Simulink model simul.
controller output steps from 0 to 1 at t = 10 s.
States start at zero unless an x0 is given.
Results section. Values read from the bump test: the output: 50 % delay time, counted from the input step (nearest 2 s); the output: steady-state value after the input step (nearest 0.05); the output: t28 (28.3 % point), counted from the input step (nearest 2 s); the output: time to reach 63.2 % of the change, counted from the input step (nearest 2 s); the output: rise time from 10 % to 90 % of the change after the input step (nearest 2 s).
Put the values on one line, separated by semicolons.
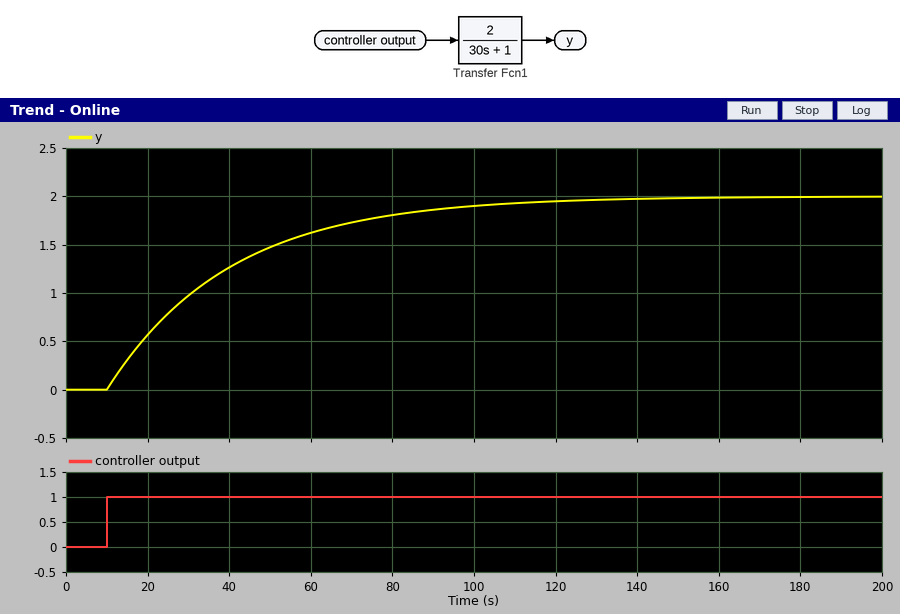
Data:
20 s; 2.00; 10 s; 30 s; 66 s
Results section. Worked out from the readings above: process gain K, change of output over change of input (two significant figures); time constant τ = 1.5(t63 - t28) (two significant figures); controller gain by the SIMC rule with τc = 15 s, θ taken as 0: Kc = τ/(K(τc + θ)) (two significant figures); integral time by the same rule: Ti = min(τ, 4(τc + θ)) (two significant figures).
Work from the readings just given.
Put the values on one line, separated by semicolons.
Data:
2.0; 30 s; 1.0; 30 s
